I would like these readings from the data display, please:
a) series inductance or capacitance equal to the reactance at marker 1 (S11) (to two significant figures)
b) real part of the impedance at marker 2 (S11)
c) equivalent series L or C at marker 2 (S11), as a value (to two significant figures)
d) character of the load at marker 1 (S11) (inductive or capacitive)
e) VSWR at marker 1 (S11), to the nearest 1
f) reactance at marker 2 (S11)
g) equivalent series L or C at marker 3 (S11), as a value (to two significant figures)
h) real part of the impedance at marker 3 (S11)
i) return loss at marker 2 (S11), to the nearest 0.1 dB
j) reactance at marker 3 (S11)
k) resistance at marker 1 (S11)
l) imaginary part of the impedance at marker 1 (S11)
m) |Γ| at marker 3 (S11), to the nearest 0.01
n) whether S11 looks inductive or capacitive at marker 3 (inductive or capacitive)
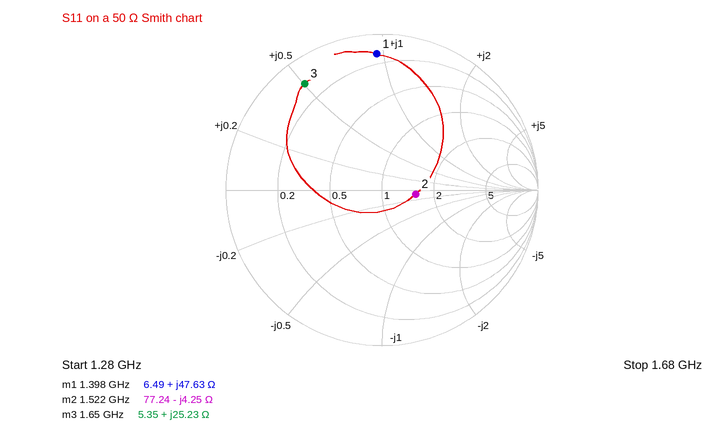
5.4 nH
77.24 Ω
25 pF
inductive
15
-4.25 Ω
2.4 nH
5.35 Ω
13.3 dB
+25.23 Ω
6.49 Ω
+47.63 Ω
0.84
inductive
